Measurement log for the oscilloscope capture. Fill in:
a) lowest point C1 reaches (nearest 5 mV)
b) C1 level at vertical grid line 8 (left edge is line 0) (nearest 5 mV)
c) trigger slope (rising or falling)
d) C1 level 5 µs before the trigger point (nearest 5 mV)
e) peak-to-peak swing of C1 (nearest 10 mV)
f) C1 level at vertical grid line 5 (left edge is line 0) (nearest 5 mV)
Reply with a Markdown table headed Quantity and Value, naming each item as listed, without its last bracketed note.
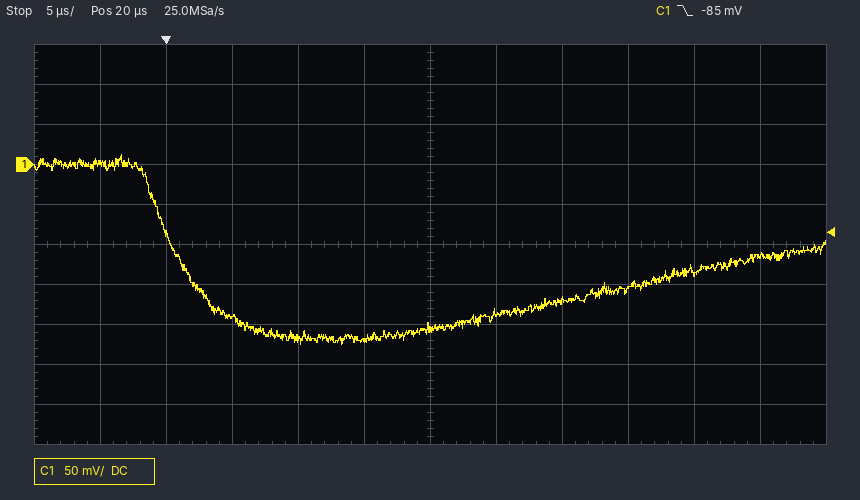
| Quantity | Value |
|---|---|
| lowest point C1 reaches | -225 mV |
| C1 level at vertical grid line 8 (left edge is line 0) | -170 mV |
| trigger slope | falling |
| C1 level 5 µs before the trigger point | 0 mV |
| peak-to-peak swing of C1 | 240 mV |
| C1 level at vertical grid line 5 (left edge is line 0) | -220 mV |
